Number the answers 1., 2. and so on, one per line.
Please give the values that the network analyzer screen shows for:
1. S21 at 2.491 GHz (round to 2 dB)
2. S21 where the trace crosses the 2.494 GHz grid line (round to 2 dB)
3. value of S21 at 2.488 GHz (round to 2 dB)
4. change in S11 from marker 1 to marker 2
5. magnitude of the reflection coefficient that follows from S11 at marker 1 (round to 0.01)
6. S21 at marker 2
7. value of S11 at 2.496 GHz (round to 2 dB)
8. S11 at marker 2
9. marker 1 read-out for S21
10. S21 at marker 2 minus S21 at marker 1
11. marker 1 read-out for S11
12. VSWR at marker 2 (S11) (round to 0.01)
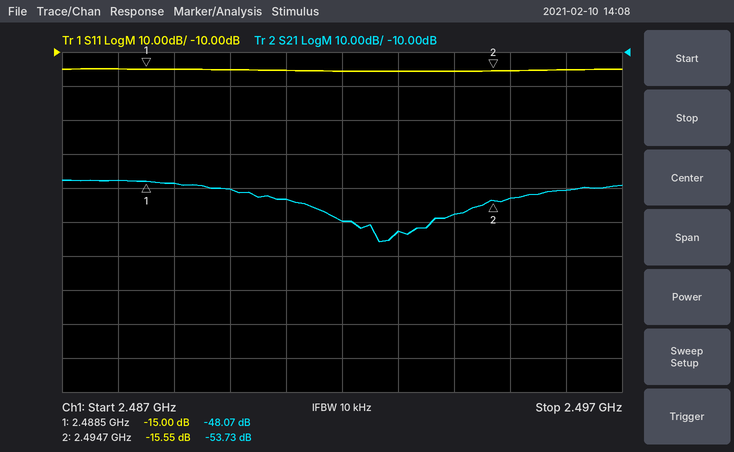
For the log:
1. -54 dB
2. -58 dB
3. -48 dB
4. -0.55 dB
5. 0.18
6. -53.73 dB
7. -16 dB
8. -15.55 dB
9. -48.07 dB
10. -5.66 dB
11. -15.00 dB
12. 1.40
